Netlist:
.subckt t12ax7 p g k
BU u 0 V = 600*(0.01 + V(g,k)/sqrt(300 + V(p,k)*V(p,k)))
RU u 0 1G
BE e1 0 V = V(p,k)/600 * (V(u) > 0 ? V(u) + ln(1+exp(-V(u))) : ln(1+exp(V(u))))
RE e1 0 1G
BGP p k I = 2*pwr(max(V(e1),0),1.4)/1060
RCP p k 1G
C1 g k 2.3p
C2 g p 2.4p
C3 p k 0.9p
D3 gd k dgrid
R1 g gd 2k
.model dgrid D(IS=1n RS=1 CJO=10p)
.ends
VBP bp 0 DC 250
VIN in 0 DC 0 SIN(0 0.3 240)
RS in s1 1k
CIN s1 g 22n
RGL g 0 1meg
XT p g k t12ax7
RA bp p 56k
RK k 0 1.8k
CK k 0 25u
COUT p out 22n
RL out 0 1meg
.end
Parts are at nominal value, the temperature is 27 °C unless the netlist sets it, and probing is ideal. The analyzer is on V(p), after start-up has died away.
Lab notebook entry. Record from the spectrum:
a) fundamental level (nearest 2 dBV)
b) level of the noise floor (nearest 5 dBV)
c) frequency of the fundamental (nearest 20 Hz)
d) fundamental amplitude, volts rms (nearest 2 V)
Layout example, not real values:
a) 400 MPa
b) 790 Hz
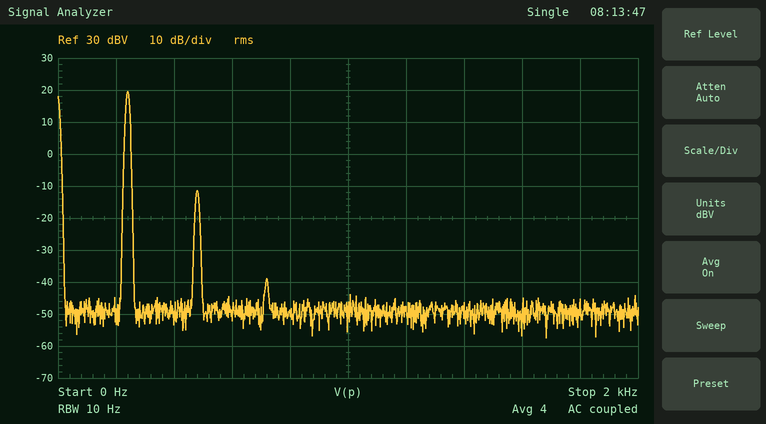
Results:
a) 20 dBV
b) -50 dBV
c) 240 Hz
d) 10 V
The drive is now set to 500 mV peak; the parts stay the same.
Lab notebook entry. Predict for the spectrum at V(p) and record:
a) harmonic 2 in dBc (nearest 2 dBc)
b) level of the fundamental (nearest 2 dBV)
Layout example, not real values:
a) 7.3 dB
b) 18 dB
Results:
a) -26 dBc
b) 24 dBV
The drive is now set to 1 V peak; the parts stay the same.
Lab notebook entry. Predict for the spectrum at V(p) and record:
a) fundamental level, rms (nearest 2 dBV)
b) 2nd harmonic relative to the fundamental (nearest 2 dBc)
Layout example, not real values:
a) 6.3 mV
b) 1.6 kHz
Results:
a) 30 dBV
b) -20 dBc
